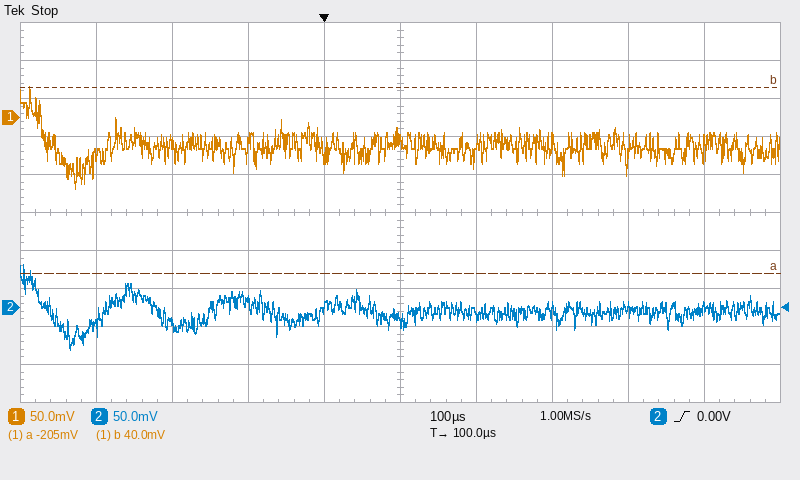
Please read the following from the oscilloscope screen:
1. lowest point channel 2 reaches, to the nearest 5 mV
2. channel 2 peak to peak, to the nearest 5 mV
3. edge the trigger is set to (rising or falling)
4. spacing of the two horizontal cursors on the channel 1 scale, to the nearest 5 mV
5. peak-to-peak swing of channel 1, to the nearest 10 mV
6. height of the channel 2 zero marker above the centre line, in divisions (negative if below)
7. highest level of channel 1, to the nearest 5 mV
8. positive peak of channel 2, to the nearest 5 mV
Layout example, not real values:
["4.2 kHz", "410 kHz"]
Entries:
["-55 mV", "110 mV", "rising", "245 mV", "130 mV", "-2.5 div", "40 mV", "55 mV"]
